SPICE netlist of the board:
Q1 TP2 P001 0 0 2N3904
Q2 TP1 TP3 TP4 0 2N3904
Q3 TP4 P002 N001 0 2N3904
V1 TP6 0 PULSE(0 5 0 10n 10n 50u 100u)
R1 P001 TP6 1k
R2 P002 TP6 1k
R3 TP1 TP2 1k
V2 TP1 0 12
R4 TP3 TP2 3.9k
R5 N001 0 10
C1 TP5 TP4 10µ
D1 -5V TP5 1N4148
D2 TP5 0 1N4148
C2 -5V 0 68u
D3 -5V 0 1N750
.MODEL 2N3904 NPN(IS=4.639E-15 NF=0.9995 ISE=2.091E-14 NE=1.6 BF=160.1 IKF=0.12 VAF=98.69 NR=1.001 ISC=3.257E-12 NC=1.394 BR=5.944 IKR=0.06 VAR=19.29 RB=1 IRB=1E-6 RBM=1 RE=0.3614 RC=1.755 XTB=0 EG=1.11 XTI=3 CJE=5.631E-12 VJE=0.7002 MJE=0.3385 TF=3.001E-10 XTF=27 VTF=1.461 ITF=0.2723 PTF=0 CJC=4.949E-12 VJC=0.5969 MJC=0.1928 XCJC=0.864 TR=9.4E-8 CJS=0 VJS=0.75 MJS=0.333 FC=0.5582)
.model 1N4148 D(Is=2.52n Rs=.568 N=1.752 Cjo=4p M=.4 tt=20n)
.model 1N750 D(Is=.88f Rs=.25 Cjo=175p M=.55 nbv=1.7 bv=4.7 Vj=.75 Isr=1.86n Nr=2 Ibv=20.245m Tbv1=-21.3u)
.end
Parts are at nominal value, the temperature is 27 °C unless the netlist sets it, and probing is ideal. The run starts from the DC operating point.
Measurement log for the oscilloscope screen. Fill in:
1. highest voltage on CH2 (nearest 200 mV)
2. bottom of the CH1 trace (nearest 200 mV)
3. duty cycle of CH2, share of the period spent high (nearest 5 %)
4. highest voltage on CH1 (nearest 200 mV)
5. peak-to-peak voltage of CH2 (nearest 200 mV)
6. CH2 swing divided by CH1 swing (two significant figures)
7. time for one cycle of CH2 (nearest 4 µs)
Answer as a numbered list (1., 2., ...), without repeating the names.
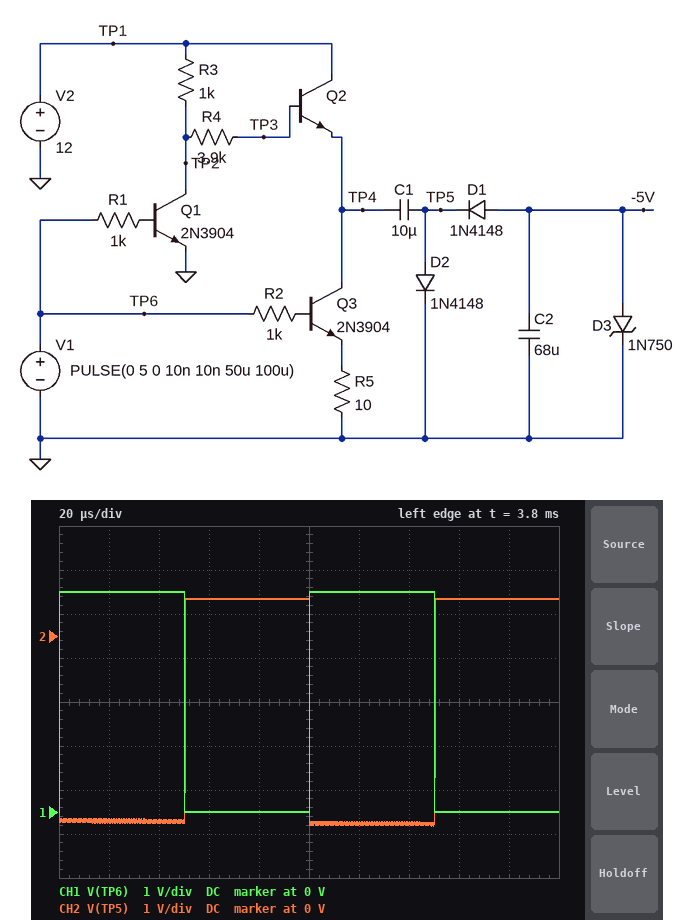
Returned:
1. 800 mV
2. 0 V
3. 50 %
4. 5.0 V
5. 5.2 V
6. 1.0
7. 100 µs
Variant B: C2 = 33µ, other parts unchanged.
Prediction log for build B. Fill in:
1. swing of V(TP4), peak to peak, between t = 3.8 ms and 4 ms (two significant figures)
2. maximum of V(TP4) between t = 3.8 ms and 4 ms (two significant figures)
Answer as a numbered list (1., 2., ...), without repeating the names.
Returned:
1. 6.8 V
2. 7.6 V
